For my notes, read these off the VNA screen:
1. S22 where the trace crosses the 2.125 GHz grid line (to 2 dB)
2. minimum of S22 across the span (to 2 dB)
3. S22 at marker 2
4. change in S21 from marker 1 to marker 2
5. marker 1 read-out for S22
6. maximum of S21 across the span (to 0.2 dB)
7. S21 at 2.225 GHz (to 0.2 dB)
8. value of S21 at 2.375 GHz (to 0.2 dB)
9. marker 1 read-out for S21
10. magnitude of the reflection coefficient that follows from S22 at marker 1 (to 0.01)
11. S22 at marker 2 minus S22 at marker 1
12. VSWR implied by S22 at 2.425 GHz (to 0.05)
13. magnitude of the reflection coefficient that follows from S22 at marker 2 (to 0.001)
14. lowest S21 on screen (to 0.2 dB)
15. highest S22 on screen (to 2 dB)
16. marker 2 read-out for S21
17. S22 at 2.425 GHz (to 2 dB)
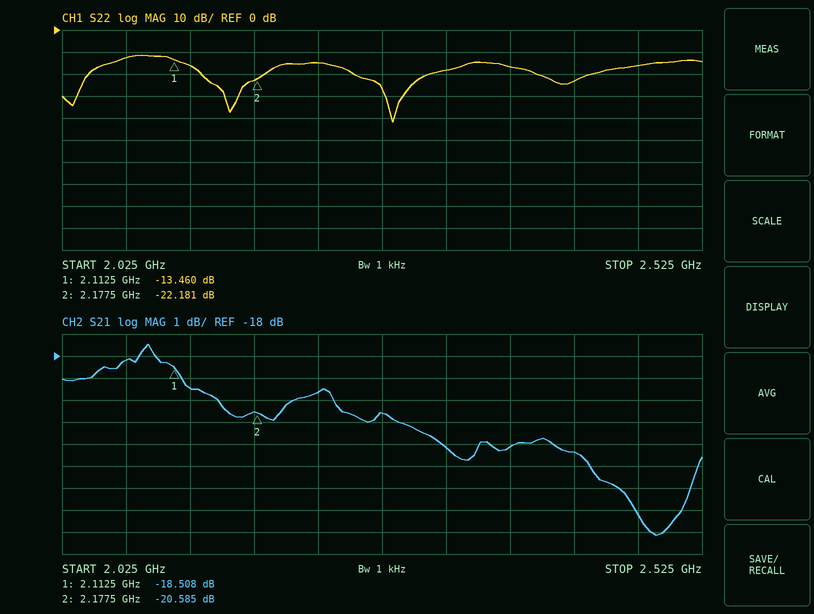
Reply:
-16 dB
-42 dB
-22.181 dB
-2.077 dB
-13.460 dB
-17.4 dB
-19.6 dB
-22.2 dB
-18.508 dB
0.21
-8.721 dB
1.15
0.078
-26.2 dB
-12 dB
-20.585 dB
-24 dB
